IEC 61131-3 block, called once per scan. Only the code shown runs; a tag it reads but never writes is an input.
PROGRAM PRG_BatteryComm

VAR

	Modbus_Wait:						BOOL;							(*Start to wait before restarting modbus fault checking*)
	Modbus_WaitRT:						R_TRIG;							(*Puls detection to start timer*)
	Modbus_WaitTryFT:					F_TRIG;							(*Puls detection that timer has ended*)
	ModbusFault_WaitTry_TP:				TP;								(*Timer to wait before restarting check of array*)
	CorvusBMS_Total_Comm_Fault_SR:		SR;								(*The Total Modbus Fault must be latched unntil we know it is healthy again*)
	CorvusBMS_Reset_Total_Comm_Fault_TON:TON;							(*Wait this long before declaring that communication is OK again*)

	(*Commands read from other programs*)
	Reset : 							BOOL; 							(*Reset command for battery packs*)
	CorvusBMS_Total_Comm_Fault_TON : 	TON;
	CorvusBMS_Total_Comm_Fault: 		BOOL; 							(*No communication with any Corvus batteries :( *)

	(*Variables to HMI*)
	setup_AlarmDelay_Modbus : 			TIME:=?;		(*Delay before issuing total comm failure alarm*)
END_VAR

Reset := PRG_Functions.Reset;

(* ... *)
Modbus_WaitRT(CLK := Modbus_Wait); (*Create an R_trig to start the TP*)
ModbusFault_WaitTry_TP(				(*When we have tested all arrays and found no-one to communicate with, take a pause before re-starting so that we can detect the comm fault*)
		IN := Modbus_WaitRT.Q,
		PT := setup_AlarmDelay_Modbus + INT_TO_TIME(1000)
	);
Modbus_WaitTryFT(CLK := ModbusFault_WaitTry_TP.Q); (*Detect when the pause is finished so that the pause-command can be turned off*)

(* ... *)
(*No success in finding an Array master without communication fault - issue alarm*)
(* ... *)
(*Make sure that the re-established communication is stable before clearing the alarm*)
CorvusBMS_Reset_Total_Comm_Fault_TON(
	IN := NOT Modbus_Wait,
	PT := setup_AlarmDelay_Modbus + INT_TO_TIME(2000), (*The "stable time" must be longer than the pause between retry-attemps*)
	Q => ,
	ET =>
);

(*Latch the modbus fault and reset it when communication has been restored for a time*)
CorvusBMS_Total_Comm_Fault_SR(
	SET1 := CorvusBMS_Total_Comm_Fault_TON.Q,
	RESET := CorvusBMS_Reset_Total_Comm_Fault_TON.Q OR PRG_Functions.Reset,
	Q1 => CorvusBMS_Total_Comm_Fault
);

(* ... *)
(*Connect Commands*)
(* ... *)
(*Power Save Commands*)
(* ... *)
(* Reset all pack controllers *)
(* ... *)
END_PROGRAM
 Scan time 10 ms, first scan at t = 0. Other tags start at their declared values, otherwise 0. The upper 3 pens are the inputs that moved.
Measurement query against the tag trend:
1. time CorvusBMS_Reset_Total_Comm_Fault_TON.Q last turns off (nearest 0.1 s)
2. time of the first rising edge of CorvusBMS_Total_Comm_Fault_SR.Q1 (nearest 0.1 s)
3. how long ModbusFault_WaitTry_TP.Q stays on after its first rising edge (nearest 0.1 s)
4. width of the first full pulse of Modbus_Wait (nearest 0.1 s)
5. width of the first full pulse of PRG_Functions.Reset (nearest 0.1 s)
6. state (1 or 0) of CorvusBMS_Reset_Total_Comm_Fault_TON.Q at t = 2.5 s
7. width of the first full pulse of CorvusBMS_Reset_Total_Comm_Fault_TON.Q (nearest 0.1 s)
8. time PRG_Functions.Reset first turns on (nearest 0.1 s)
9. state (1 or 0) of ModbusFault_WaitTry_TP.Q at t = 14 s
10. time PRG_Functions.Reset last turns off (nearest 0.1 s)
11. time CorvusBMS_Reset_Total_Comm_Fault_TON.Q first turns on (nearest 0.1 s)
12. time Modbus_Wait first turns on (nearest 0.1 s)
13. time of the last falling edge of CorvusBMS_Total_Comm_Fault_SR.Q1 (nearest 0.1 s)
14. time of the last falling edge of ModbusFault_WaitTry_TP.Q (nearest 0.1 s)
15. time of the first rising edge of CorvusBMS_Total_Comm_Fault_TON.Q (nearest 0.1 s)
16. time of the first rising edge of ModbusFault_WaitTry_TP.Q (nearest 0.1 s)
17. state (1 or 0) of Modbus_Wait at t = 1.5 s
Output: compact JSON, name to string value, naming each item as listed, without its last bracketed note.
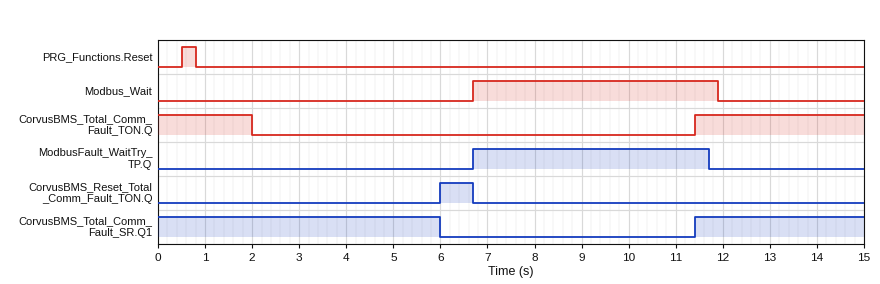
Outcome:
{"time CorvusBMS_Reset_Total_Comm_Fault_TON.Q last turns off": "6.7 s", "time of the first rising edge of CorvusBMS_Total_Comm_Fault_SR.Q1": "11.4 s", "how long ModbusFault_WaitTry_TP.Q stays on after its first rising edge": "5.0 s", "width of the first full pulse of Modbus_Wait": "5.2 s", "width of the first full pulse of PRG_Functions.Reset": "0.3 s", "state (1 or 0) of CorvusBMS_Reset_Total_Comm_Fault_TON.Q at t = 2.5 s": "0", "width of the first full pulse of CorvusBMS_Reset_Total_Comm_Fault_TON.Q": "0.7 s", "time PRG_Functions.Reset first turns on": "0.5 s", "state (1 or 0) of ModbusFault_WaitTry_TP.Q at t = 14 s": "0", "time PRG_Functions.Reset last turns off": "0.8 s", "time CorvusBMS_Reset_Total_Comm_Fault_TON.Q first turns on": "6.0 s", "time Modbus_Wait first turns on": "6.7 s", "time of the last falling edge of CorvusBMS_Total_Comm_Fault_SR.Q1": "6.0 s", "time of the last falling edge of ModbusFault_WaitTry_TP.Q": "11.7 s", "time of the first rising edge of CorvusBMS_Total_Comm_Fault_TON.Q": "11.4 s", "time of the first rising edge of ModbusFault_WaitTry_TP.Q": "6.7 s", "state (1 or 0) of Modbus_Wait at t = 1.5 s": "0"}
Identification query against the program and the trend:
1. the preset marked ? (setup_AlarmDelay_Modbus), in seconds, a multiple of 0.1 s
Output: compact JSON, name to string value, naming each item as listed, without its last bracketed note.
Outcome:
{"the preset marked ? (setup_AlarmDelay_Modbus), in seconds, a multiple of 0.1 s": "4.0 s"}
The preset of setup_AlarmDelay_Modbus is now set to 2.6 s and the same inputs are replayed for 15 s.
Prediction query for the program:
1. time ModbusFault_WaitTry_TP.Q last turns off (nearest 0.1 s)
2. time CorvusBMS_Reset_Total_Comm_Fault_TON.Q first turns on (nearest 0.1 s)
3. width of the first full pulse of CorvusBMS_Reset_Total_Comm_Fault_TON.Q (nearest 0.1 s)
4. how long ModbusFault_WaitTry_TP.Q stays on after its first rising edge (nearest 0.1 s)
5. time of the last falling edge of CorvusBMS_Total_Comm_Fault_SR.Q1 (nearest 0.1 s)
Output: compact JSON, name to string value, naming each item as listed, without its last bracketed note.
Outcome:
{"time ModbusFault_WaitTry_TP.Q last turns off": "10.3 s", "time CorvusBMS_Reset_Total_Comm_Fault_TON.Q first turns on": "4.6 s", "width of the first full pulse of CorvusBMS_Reset_Total_Comm_Fault_TON.Q": "2.1 s", "how long ModbusFault_WaitTry_TP.Q stays on after its first rising edge": "3.6 s", "time of the last falling edge of CorvusBMS_Total_Comm_Fault_SR.Q1": "4.6 s"}
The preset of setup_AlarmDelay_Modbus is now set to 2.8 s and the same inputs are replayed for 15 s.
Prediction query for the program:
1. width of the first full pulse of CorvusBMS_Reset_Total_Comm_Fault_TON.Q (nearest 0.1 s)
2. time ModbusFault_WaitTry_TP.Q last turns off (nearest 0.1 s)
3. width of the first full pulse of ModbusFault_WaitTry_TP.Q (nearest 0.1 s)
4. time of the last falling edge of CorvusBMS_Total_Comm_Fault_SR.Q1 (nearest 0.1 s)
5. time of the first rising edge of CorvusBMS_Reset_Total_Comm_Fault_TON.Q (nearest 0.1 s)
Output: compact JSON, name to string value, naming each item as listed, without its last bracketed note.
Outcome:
{"width of the first full pulse of CorvusBMS_Reset_Total_Comm_Fault_TON.Q": "1.9 s", "time ModbusFault_WaitTry_TP.Q last turns off": "10.5 s", "width of the first full pulse of ModbusFault_WaitTry_TP.Q": "3.8 s", "time of the last falling edge of CorvusBMS_Total_Comm_Fault_SR.Q1": "4.8 s", "time of the first rising edge of CorvusBMS_Reset_Total_Comm_Fault_TON.Q": "4.8 s"}
